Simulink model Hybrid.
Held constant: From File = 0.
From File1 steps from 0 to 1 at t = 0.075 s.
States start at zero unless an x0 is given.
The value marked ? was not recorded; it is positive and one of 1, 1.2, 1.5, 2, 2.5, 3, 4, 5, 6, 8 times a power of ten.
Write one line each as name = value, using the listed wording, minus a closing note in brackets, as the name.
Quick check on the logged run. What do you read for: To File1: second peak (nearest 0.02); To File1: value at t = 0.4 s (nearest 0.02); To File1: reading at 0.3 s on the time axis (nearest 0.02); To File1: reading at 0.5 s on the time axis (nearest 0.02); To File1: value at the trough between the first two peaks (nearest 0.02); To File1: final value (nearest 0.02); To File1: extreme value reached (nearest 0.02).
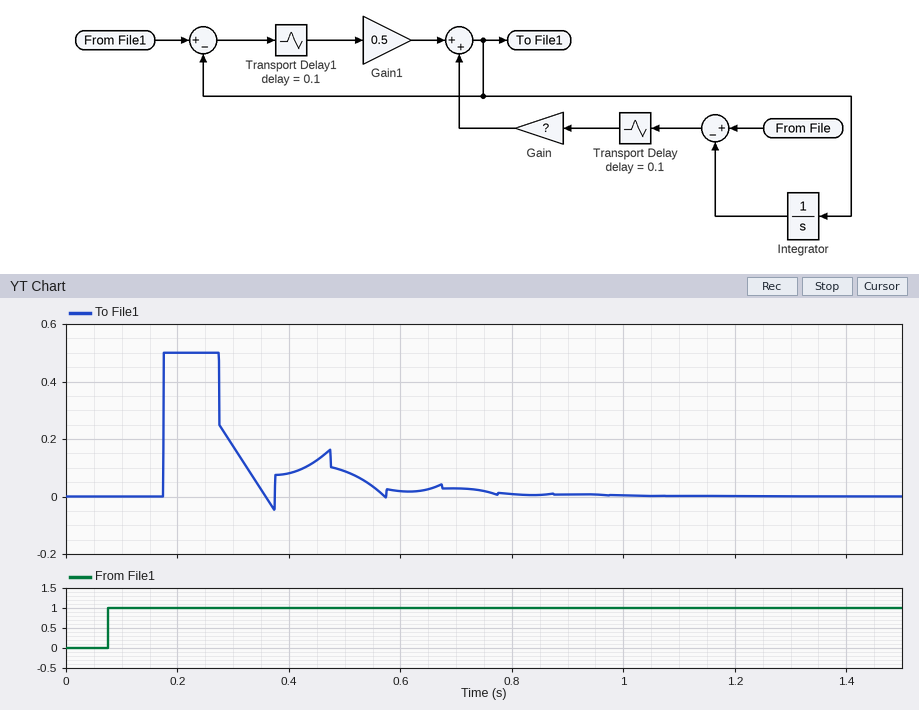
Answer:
To File1: second peak = 0.16
To File1: value at t = 0.4 s = 0.08
To File1: reading at 0.3 s on the time axis = 0.18
To File1: reading at 0.5 s on the time axis = 0.08
To File1: value at the trough between the first two peaks = -0.04
To File1: final value = 0.00
To File1: extreme value reached = 0.50
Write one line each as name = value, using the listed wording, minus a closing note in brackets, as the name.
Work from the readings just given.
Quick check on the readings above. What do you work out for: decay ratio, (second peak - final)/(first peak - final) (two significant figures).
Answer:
decay ratio, (second peak - final)/(first peak - final) = 0.32
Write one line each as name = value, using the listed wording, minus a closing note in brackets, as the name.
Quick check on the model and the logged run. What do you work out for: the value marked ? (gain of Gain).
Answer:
the value marked ? = 6
